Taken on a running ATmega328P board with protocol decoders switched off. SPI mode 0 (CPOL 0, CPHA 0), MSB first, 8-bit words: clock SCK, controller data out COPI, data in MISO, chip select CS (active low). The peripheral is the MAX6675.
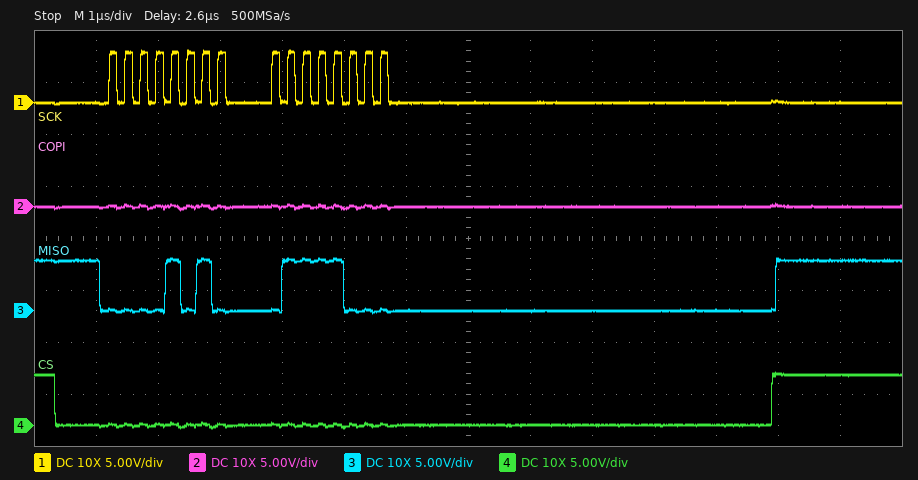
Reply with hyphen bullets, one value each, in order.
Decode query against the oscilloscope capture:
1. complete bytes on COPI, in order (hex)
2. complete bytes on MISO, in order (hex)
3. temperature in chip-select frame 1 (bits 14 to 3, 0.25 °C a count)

- 0x00 0x00
- 0x0A 0x78
- 83.75 °C
